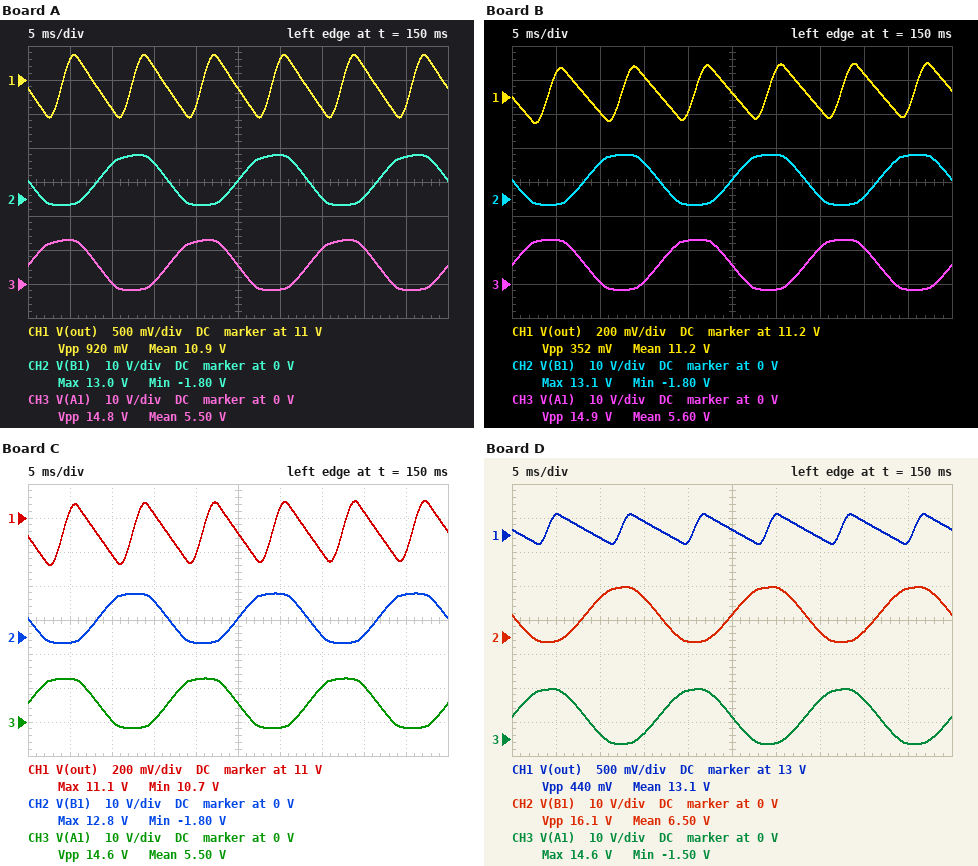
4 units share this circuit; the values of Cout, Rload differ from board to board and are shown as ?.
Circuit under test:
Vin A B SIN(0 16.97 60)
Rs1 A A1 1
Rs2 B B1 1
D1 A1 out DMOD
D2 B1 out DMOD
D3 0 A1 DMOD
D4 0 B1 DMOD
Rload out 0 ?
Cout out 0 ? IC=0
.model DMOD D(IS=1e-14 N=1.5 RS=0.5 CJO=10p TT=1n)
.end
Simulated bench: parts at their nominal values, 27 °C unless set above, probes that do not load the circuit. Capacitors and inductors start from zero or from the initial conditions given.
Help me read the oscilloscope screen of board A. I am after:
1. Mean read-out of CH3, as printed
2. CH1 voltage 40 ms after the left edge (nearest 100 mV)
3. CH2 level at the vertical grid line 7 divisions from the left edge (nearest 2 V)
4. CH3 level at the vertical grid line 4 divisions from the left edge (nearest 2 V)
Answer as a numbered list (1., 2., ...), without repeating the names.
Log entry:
1. 5.50 V
2. 11.2 V
3. 0 V
4. 12 V
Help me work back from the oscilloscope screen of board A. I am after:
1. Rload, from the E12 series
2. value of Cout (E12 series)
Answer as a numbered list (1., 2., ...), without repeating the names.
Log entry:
1. 33 Ω
2. 1.8 mF
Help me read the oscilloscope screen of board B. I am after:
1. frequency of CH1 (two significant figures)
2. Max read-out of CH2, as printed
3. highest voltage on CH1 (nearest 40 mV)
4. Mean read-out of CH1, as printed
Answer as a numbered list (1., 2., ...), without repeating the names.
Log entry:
1. 120 Hz
2. 13.1 V
3. 11.40 V
4. 11.2 V
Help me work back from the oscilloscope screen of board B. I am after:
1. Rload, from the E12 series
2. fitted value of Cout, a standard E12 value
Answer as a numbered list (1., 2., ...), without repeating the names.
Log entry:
1. 39 Ω
2. 4.7 mF
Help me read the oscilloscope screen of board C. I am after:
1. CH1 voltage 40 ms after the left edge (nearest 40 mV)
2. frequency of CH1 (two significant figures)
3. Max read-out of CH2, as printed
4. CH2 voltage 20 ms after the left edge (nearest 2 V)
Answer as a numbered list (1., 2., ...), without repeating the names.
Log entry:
1. 11.04 V
2. 120 Hz
3. 12.8 V
4. -2 V
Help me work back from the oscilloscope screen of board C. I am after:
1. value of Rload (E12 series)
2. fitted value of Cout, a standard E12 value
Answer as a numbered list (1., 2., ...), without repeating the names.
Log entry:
1. 33 Ω
2. 4.7 mF
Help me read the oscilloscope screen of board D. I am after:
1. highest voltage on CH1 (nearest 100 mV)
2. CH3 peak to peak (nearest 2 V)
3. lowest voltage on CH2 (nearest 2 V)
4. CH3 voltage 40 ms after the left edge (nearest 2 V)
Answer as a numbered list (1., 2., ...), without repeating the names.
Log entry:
1. 13.3 V
2. 16 V
3. -2 V
4. 12 V
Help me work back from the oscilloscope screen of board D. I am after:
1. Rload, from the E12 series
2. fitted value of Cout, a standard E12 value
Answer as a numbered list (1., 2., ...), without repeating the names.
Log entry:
1. 150 Ω
2. 1.2 mF
